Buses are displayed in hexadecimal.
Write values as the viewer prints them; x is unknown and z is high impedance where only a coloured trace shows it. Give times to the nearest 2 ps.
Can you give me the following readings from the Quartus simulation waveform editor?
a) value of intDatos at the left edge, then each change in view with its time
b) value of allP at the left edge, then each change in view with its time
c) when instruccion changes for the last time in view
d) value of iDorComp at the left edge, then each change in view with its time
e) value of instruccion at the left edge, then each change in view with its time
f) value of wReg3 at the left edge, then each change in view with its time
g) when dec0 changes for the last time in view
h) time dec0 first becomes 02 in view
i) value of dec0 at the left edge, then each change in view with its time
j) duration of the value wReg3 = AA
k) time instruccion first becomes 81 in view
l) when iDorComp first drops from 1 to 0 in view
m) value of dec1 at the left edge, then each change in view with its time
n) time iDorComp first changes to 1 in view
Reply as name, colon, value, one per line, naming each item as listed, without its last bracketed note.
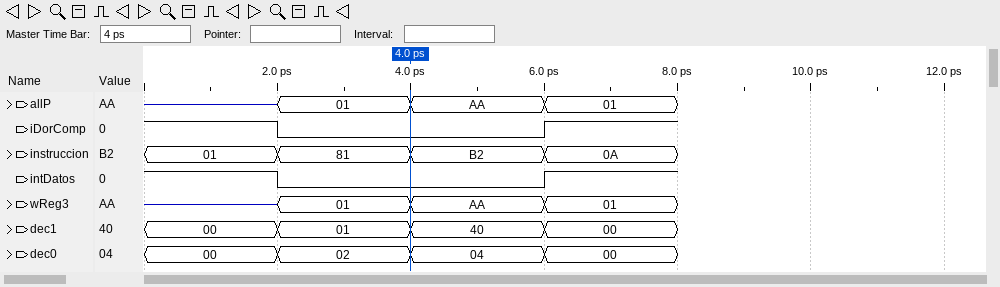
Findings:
value of intDatos at the left edge, then each change in view with its time: 1, 0 at 2 ps, 1 at 6 ps
value of allP at the left edge, then each change in view with its time: z, 01 at 2 ps, AA at 4 ps, 01 at 6 ps
when instruccion changes for the last time in view: 6 ps
value of iDorComp at the left edge, then each change in view with its time: 1, 0 at 2 ps, 1 at 6 ps
value of instruccion at the left edge, then each change in view with its time: 01, 81 at 2 ps, B2 at 4 ps, 0A at 6 ps
value of wReg3 at the left edge, then each change in view with its time: z, 01 at 2 ps, AA at 4 ps, 01 at 6 ps
when dec0 changes for the last time in view: 6 ps
time dec0 first becomes 02 in view: 2 ps
value of dec0 at the left edge, then each change in view with its time: 00, 02 at 2 ps, 04 at 4 ps, 00 at 6 ps
duration of the value wReg3 = AA: 2 ps
time instruccion first becomes 81 in view: 2 ps
when iDorComp first drops from 1 to 0 in view: 2 ps
value of dec1 at the left edge, then each change in view with its time: 00, 01 at 2 ps, 40 at 4 ps, 00 at 6 ps
time iDorComp first changes to 1 in view: 6 ps
